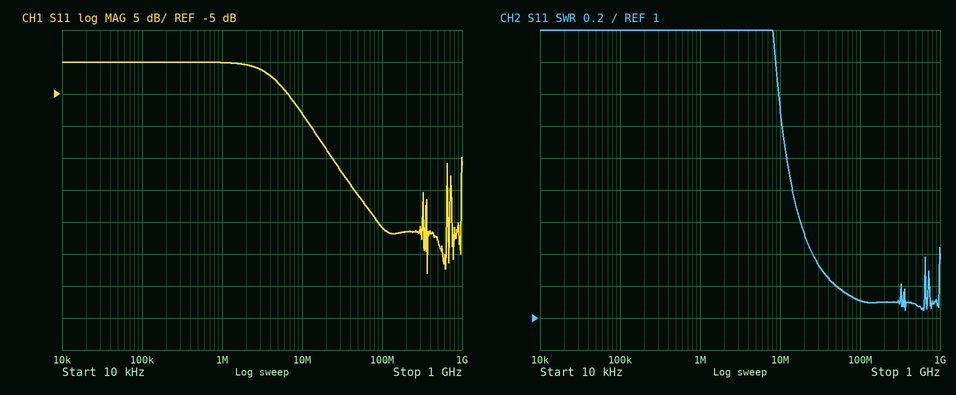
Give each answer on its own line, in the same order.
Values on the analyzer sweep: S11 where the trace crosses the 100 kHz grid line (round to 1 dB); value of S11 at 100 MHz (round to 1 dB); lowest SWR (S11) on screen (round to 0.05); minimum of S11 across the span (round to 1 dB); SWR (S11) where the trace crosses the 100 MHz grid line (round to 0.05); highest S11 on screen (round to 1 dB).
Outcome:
0 dB
-26 dB
1.05
-33 dB
1.10
0 dB
